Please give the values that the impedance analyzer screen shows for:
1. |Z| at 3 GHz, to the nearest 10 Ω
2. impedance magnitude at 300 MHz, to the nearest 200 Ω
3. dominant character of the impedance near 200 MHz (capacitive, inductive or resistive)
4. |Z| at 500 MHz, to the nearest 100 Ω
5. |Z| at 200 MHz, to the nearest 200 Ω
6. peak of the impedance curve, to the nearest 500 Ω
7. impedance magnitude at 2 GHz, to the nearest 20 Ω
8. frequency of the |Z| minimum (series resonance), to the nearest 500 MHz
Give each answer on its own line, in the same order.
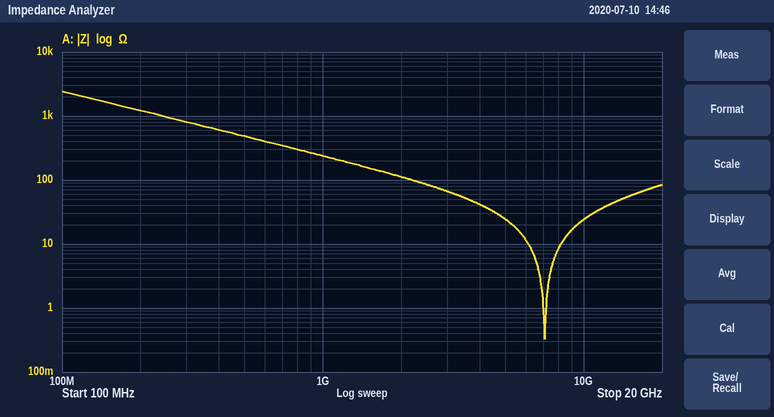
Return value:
70 Ω
800 Ω
capacitive
500 Ω
1.2 kΩ
2.5 kΩ
120 Ω
7.0 GHz
